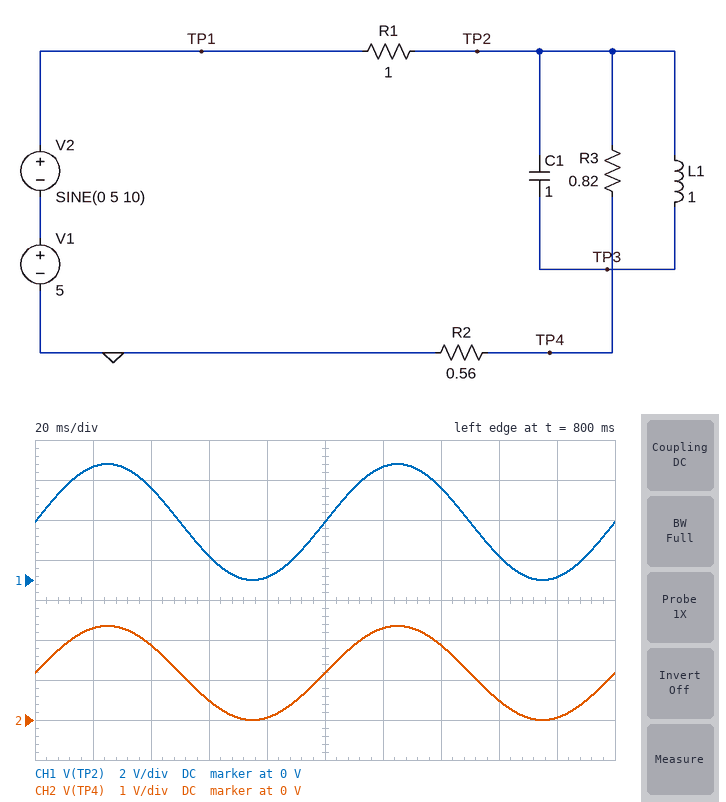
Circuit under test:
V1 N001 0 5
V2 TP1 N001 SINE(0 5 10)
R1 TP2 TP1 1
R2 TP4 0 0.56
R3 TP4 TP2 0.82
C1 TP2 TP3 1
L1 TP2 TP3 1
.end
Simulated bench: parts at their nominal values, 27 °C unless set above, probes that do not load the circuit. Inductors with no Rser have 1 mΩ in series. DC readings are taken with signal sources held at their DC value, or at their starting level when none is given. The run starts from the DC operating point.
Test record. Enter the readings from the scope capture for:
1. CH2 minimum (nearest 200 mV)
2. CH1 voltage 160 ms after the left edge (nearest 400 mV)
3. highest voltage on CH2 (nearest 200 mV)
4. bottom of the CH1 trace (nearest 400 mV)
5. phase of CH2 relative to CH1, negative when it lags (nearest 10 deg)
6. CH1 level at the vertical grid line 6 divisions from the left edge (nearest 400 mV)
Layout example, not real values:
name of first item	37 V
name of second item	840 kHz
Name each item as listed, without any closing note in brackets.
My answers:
CH2 minimum	0 V
CH1 voltage 160 ms after the left edge	1.2 V
highest voltage on CH2	2.4 V
bottom of the CH1 trace	0 V
phase of CH2 relative to CH1, negative when it lags	0 deg
CH1 level at the vertical grid line 6 divisions from the left edge	5.6 V
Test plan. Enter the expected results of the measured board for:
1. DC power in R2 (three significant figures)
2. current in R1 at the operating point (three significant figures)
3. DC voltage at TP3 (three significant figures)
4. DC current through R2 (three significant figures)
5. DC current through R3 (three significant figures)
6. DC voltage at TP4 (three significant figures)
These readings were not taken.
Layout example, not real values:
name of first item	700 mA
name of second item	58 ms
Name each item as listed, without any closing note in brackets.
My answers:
DC power in R2	2.47 W
current in R1 at the operating point	2.10 A
DC voltage at TP3	2.90 V
DC current through R2	2.10 A
DC current through R3	2.10 A
DC voltage at TP4	1.18 V
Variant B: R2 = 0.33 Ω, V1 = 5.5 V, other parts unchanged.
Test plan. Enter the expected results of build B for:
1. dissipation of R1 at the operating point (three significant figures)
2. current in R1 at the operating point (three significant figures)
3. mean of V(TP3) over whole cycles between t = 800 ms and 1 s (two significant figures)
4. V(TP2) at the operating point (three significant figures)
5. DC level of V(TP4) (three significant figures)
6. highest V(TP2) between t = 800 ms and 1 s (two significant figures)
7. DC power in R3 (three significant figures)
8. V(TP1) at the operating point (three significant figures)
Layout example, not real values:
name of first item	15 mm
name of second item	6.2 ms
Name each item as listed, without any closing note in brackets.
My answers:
dissipation of R1 at the operating point	6.54 W
current in R1 at the operating point	2.56 A
mean of V(TP3) over whole cycles between t = 800 ms and 1 s	2.9 V
V(TP2) at the operating point	2.94 V
DC level of V(TP4)	844 mV
highest V(TP2) between t = 800 ms and 1 s	5.6 V
DC power in R3	5.37 W
V(TP1) at the operating point	5.50 V
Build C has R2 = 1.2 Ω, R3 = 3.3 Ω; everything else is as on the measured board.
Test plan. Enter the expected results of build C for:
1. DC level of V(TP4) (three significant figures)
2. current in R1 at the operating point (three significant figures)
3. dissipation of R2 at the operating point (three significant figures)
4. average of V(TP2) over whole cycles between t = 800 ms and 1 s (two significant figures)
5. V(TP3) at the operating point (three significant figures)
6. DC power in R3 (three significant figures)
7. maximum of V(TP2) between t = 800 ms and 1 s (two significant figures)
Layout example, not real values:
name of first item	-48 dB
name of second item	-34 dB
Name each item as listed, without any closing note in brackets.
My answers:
DC level of V(TP4)	1.09 V
current in R1 at the operating point	909 mA
dissipation of R2 at the operating point	992 mW
average of V(TP2) over whole cycles between t = 800 ms and 1 s	4.1 V
V(TP3) at the operating point	4.09 V
DC power in R3	2.73 W
maximum of V(TP2) between t = 800 ms and 1 s	8.2 V
